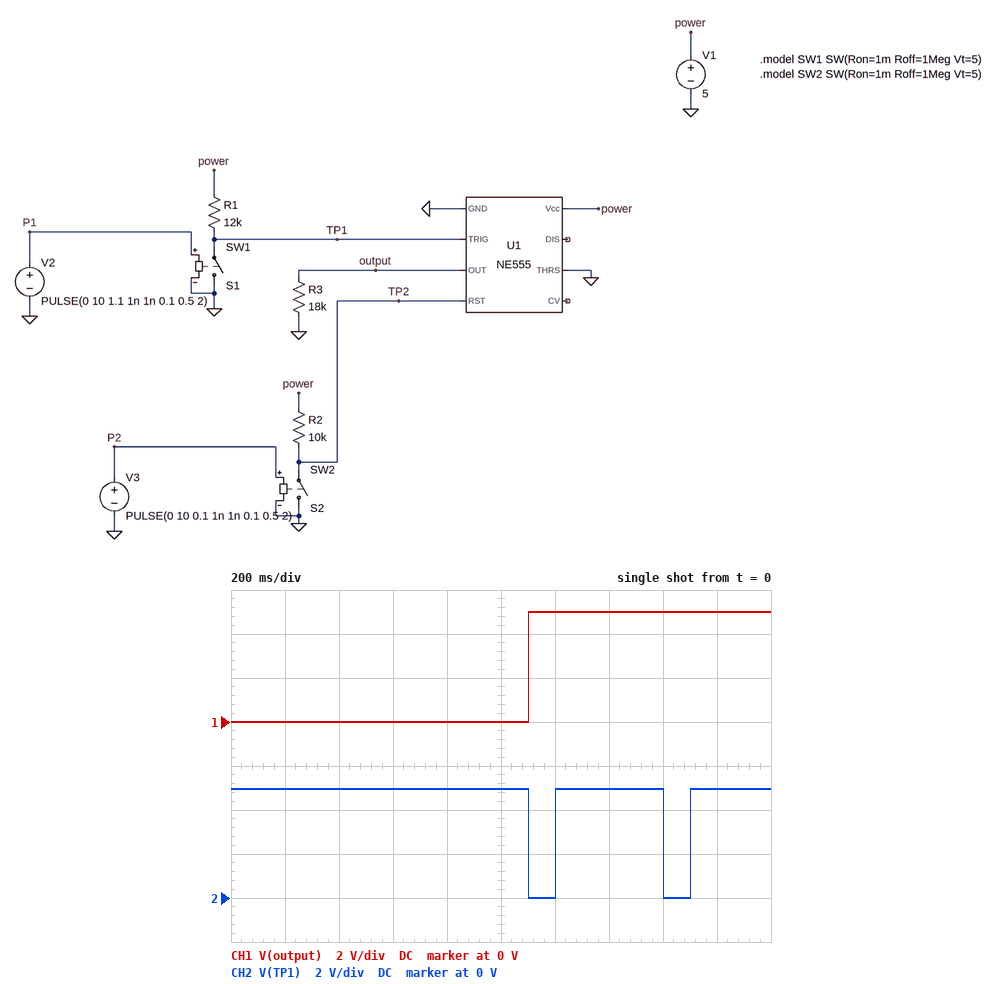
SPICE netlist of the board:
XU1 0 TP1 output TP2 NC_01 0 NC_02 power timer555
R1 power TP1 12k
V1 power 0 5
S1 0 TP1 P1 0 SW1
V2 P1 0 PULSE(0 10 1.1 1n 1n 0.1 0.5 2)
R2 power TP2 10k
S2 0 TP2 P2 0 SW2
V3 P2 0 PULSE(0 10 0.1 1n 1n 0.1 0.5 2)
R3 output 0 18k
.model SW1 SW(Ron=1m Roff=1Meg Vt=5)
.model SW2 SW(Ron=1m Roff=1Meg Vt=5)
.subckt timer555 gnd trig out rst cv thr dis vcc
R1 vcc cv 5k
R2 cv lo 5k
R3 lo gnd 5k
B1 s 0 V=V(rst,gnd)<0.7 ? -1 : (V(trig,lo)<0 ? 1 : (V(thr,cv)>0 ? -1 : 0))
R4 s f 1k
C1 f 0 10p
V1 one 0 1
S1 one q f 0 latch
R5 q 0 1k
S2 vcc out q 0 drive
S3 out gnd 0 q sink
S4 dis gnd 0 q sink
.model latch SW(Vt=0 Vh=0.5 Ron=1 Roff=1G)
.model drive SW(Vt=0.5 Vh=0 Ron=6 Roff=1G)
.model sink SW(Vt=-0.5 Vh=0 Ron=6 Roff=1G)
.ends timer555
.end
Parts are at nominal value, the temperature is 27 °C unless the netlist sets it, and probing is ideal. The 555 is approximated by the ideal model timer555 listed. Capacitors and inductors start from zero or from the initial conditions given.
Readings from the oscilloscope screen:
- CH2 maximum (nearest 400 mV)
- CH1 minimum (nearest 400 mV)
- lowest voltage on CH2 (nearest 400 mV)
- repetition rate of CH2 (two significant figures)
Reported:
4.8 V
0 V
0 V
2.0 Hz
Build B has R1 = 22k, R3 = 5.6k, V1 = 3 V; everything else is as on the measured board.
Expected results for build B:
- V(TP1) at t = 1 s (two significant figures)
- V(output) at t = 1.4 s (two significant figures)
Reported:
2.9 V
3.0 V
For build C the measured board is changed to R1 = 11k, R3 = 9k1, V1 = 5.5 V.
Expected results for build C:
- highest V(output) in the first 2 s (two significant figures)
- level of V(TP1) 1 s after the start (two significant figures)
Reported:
5.5 V
5.4 V
